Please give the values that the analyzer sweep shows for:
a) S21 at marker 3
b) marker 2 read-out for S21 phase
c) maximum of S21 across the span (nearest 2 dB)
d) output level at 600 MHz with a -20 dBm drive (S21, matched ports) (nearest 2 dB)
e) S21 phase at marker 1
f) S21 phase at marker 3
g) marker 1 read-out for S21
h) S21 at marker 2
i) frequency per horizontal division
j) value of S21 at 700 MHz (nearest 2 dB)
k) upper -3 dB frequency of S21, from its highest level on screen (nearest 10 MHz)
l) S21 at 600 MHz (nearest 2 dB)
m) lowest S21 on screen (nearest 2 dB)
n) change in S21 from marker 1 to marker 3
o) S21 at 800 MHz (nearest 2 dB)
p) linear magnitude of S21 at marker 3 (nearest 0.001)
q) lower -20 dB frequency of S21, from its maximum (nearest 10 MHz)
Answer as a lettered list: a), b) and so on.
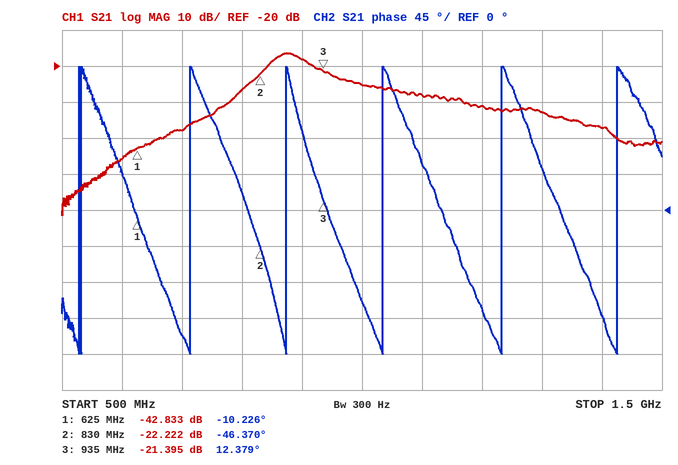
a) -21.395 dB
b) -46.370°
c) -16 dB
d) -66 dBm
e) -10.226°
f) 12.379°
g) -42.833 dB
h) -22.222 dB
i) 100 MHz
j) -38 dB
k) 910 MHz
l) -46 dB
m) -62 dB
n) 21.438 dB
o) -26 dB
p) 0.085
q) 710 MHz
